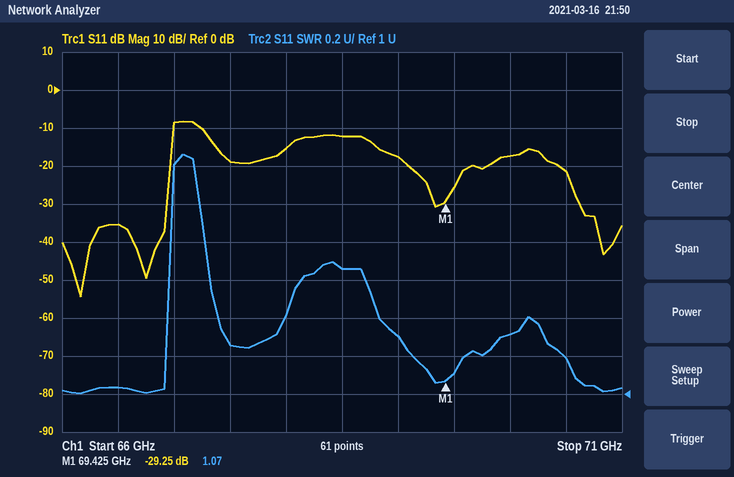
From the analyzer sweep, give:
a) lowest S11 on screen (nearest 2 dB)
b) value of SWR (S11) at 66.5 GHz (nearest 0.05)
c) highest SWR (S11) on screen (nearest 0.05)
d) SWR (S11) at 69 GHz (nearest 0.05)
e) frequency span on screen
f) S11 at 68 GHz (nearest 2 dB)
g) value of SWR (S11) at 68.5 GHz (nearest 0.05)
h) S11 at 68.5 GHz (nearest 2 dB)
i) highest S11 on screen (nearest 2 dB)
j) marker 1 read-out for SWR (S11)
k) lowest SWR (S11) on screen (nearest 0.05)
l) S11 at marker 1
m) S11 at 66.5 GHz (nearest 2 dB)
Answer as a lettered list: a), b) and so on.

a) -54 dB
b) 1.05
c) 2.25
d) 1.30
e) 5 GHz
f) -16 dB
g) 1.65
h) -12 dB
i) -8 dB
j) 1.07
k) 1.00
l) -29.25 dB
m) -36 dB
